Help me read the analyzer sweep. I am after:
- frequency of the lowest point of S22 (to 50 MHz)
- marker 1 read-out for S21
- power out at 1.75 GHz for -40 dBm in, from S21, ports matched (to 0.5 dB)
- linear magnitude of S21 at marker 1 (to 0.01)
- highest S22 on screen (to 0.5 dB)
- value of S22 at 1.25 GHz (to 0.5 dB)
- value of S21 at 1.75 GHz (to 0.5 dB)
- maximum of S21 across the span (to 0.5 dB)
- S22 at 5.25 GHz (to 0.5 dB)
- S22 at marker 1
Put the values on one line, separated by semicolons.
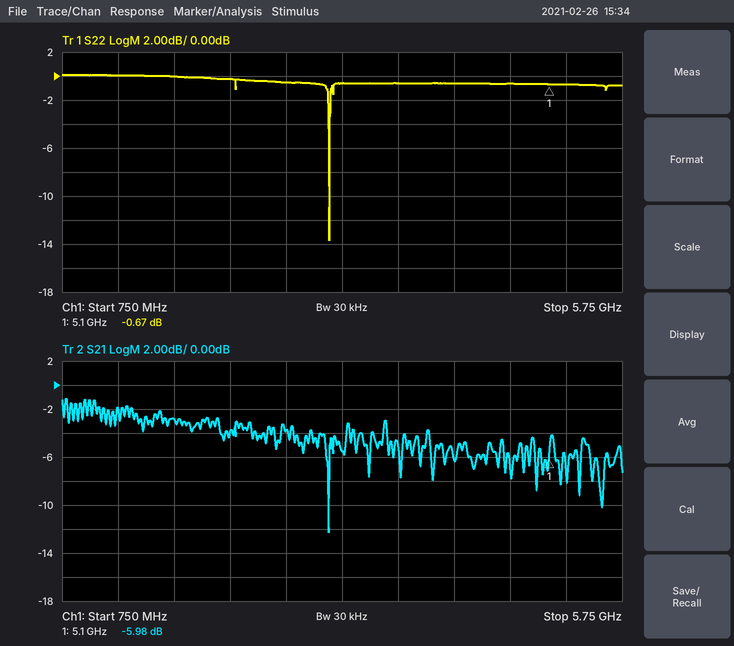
3.15 GHz; -5.98 dB; -43.0 dBm; 0.50; 0.0 dB; 0.0 dB; -3.0 dB; -1.0 dB; -0.5 dB; -0.67 dB
